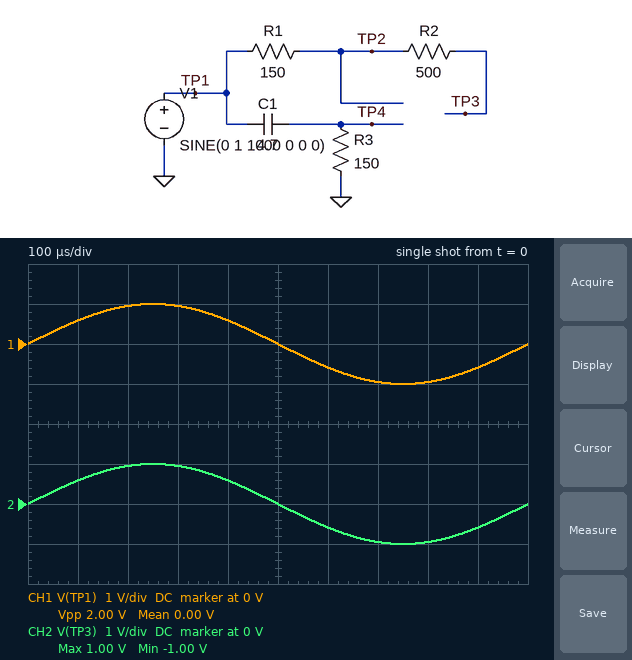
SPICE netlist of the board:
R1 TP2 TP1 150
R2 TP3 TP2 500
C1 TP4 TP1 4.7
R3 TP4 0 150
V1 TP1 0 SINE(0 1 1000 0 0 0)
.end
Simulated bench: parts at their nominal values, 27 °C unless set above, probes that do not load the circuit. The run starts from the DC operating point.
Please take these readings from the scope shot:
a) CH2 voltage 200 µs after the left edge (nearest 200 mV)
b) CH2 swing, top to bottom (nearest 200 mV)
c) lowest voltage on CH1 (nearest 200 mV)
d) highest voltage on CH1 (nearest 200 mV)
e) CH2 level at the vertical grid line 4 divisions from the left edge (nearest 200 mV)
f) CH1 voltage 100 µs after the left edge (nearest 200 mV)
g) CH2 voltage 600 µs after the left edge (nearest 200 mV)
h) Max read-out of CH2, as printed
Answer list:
1.0 V
2.0 V
-1.0 V
1.0 V
600 mV
600 mV
-600 mV
1.00 V
